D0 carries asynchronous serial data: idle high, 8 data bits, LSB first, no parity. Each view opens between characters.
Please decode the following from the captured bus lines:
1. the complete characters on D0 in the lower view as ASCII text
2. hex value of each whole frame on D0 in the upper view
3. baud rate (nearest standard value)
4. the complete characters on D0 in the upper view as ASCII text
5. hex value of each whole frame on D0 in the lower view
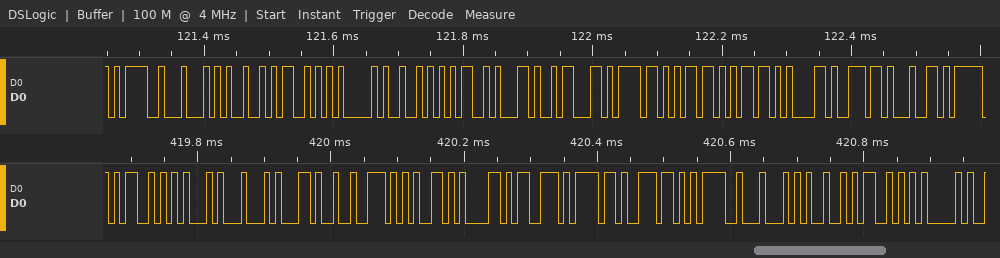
"MED,reason=DISA"
3D, 44, 49, 53, 41, 52, 4D, 2C, 63, 6F, 6D, 6D, 61, 6E, 64
115200 baud
"=DISARM,command"
4D, 45, 44, 2C, 72, 65, 61, 73, 6F, 6E, 3D, 44, 49, 53, 41
